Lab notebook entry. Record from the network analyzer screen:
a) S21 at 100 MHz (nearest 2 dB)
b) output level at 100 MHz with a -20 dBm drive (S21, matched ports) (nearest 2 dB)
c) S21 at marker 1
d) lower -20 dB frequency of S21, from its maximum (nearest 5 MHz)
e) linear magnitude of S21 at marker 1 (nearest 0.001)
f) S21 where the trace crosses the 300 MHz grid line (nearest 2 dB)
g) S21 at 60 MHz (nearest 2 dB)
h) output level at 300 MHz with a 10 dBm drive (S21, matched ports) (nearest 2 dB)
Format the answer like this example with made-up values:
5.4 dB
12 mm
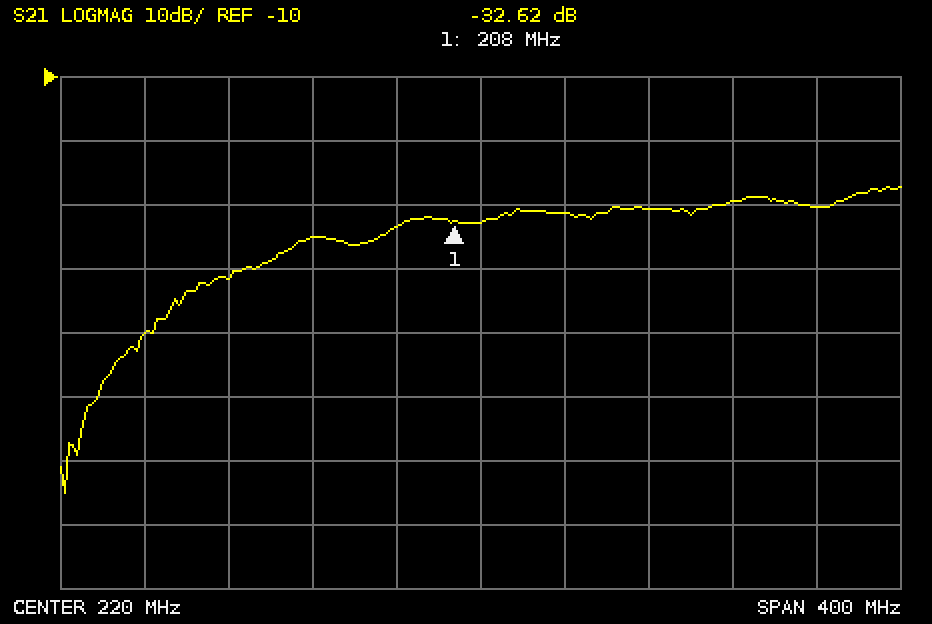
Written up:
-42 dB
-62 dBm
-32.62 dB
70 MHz
0.023
-30 dB
-50 dB
-20 dBm
